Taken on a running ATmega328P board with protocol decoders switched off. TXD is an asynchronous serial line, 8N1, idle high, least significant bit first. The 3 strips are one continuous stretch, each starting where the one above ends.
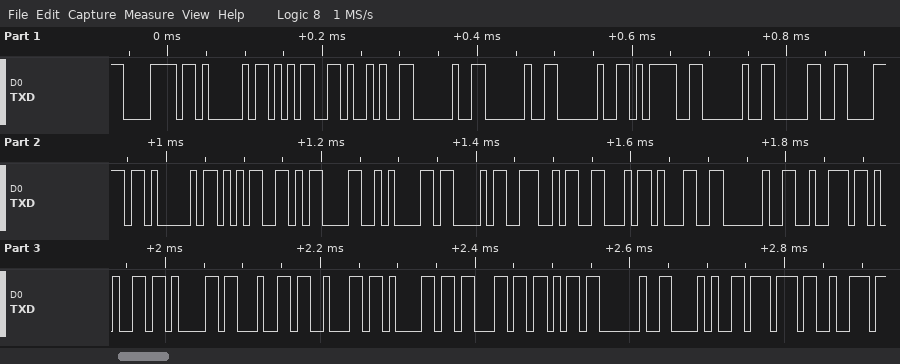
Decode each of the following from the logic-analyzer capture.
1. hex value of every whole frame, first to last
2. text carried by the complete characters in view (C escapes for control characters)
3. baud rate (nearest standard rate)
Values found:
78 41 35 29 20 20 20 3D 20 30 78 41 35 0D 0A 43 4E 46 31 20 72 65 61 64 62 61 63 6B 20 28 77 72
"xA5)   = 0xA5\r\nCNF1 readback (wr"
115200 baud
